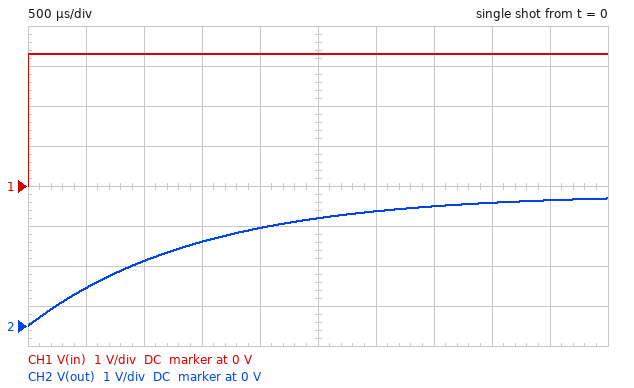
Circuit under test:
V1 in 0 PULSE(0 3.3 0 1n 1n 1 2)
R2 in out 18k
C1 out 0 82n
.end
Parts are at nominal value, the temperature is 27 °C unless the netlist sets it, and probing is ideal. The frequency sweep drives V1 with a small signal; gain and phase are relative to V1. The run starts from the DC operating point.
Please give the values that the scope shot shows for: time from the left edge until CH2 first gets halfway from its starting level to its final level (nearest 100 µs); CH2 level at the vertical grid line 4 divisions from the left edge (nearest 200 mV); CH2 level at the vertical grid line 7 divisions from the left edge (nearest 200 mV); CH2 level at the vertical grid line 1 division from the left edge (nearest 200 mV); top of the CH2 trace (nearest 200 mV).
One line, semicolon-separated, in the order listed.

1.0 ms; 2.4 V; 3.0 V; 1.0 V; 3.2 V
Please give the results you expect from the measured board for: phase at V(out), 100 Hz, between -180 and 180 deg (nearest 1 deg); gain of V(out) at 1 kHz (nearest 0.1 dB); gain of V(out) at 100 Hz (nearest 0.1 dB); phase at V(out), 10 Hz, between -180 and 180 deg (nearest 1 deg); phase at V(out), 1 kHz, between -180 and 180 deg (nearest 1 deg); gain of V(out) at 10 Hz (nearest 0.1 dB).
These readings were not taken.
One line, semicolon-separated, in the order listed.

-43 deg; -19.4 dB; -2.7 dB; -5 deg; -84 deg; 0 dB
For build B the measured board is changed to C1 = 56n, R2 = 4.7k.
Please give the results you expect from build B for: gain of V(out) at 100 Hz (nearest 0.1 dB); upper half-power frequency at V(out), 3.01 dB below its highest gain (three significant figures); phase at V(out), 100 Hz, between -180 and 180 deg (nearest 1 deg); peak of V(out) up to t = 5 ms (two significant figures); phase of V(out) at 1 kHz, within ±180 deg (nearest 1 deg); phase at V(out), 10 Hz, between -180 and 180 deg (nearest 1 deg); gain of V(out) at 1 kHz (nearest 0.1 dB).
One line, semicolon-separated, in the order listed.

-0.1 dB; 605 Hz; -9 deg; 3.3 V; -59 deg; -1 deg; -5.7 dB
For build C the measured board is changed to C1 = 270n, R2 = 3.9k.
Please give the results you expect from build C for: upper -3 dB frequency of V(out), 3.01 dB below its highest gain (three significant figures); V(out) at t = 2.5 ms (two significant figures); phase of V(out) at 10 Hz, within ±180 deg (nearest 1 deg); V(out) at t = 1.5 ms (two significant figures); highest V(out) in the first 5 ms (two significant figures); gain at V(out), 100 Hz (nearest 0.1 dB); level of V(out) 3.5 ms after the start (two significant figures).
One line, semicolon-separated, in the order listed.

151 Hz; 3.0 V; -4 deg; 2.5 V; 3.3 V; -1.6 dB; 3.2 V
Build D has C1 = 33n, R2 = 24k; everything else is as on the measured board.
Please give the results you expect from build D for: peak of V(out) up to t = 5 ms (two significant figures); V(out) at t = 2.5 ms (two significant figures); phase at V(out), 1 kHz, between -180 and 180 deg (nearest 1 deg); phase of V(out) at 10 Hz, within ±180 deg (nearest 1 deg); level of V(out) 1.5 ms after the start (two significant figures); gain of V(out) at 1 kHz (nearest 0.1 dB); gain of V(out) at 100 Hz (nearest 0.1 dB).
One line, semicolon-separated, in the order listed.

3.3 V; 3.2 V; -79 deg; -3 deg; 2.8 V; -14.1 dB; -1.0 dB
